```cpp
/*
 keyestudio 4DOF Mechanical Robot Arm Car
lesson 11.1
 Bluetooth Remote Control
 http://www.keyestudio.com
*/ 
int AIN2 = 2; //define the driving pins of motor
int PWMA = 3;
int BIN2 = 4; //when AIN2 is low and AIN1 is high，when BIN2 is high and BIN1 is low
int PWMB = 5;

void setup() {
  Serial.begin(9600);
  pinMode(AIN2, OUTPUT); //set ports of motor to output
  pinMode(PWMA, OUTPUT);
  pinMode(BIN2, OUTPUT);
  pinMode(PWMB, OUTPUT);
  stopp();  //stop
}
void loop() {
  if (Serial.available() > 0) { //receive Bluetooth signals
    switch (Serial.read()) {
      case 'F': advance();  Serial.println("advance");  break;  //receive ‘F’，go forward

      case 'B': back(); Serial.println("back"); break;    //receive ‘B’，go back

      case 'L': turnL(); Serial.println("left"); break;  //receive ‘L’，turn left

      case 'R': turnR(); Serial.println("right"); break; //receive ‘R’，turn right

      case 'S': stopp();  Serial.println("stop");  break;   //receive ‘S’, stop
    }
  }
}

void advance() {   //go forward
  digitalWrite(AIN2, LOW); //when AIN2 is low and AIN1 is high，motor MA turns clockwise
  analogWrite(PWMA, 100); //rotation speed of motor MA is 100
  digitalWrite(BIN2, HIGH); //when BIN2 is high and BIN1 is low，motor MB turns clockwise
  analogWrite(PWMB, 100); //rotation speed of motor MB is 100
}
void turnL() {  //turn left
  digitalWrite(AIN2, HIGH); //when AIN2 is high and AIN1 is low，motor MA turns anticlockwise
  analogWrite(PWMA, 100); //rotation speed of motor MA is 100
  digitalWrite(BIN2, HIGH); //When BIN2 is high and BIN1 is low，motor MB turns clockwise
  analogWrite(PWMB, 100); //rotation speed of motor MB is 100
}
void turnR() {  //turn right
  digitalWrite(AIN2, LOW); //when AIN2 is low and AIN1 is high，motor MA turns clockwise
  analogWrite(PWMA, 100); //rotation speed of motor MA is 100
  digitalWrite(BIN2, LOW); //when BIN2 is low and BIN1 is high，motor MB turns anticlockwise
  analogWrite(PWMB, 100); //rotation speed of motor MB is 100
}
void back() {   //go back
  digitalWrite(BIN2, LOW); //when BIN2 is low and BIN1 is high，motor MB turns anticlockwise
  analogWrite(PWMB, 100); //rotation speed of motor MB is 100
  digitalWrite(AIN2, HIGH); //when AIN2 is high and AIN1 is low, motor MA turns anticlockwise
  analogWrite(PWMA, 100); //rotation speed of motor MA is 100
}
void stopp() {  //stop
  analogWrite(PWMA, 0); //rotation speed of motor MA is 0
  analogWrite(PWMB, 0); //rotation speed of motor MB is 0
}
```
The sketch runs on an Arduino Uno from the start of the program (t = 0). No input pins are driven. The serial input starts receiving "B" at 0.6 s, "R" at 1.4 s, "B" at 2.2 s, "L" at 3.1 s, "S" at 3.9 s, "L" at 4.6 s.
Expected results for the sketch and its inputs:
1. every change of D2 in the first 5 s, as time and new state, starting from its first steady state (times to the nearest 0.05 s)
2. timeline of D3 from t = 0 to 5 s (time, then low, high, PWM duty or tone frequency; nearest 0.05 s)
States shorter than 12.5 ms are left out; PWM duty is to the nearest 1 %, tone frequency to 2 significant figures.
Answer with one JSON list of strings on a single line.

["0 s low; 0.6 s high; 1.4 s low; 2.2 s high", "0 s low; 0.6 s PWM 39 %; 3.9 s low; 4.6 s PWM 39 %"]
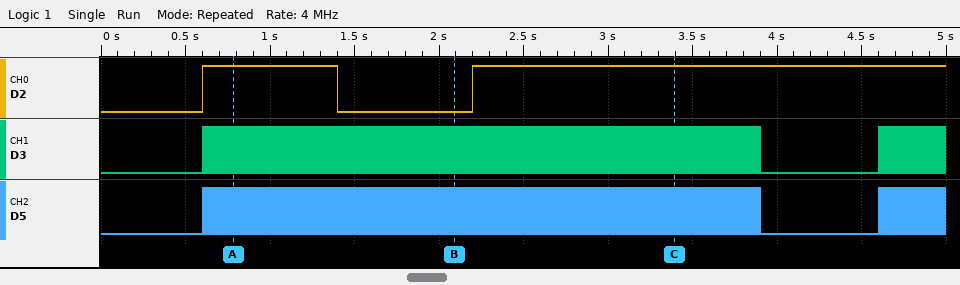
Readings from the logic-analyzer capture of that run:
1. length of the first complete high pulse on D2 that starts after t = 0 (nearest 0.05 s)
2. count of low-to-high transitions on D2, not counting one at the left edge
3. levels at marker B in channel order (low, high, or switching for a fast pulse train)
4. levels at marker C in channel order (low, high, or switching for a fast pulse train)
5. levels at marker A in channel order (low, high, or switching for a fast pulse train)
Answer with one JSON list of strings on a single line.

["0.80 s", "2", "D2 low, D3 switching, D5 switching", "D2 high, D3 switching, D5 switching", "D2 high, D3 switching, D5 switching"]
